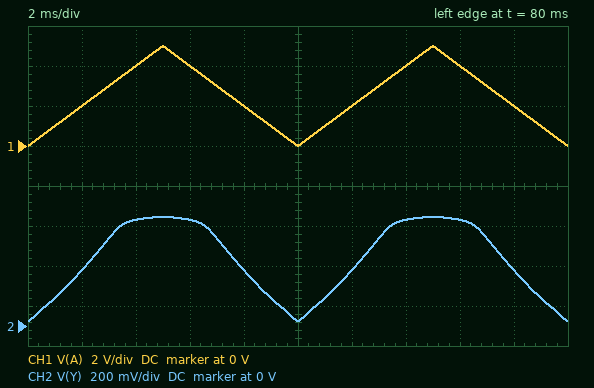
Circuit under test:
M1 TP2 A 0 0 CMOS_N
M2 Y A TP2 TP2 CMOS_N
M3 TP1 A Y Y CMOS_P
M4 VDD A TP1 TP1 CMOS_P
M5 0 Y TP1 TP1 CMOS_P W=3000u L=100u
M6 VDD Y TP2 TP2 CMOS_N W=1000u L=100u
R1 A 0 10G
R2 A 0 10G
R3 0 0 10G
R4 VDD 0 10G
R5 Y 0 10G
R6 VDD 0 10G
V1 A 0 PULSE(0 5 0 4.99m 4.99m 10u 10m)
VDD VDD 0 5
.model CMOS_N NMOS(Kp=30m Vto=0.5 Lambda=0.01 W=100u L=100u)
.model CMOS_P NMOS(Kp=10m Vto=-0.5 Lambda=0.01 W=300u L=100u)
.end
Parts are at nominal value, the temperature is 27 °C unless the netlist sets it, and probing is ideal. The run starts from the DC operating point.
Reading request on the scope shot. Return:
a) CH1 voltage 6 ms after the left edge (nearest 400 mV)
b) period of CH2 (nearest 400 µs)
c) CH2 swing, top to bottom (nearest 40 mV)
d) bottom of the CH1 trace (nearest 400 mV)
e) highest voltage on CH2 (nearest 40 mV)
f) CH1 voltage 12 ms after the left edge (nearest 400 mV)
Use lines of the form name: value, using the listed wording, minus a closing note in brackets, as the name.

CH1 voltage 6 ms after the left edge: 4.0 V
period of CH2: 10.0 ms
CH2 swing, top to bottom: 520 mV
bottom of the CH1 trace: 0 V
highest voltage on CH2: 560 mV
CH1 voltage 12 ms after the left edge: 2.0 V
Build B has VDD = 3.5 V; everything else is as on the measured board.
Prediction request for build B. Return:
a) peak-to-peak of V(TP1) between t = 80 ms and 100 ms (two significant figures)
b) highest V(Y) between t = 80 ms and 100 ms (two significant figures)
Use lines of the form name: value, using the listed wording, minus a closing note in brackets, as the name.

peak-to-peak of V(TP1) between t = 80 ms and 100 ms: 750 mV
highest V(Y) between t = 80 ms and 100 ms: 540 mV
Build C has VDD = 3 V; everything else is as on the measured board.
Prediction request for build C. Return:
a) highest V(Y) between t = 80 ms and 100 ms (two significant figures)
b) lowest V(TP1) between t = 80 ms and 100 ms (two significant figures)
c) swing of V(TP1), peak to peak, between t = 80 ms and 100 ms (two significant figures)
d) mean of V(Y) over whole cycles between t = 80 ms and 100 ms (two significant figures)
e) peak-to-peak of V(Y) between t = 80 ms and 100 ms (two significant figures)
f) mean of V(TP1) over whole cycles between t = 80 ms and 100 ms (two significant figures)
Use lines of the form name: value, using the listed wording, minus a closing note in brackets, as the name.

highest V(Y) between t = 80 ms and 100 ms: 530 mV
lowest V(TP1) between t = 80 ms and 100 ms: 23 mV
swing of V(TP1), peak to peak, between t = 80 ms and 100 ms: 740 mV
mean of V(Y) over whole cycles between t = 80 ms and 100 ms: 330 mV
peak-to-peak of V(Y) between t = 80 ms and 100 ms: 510 mV
mean of V(TP1) over whole cycles between t = 80 ms and 100 ms: 450 mV
